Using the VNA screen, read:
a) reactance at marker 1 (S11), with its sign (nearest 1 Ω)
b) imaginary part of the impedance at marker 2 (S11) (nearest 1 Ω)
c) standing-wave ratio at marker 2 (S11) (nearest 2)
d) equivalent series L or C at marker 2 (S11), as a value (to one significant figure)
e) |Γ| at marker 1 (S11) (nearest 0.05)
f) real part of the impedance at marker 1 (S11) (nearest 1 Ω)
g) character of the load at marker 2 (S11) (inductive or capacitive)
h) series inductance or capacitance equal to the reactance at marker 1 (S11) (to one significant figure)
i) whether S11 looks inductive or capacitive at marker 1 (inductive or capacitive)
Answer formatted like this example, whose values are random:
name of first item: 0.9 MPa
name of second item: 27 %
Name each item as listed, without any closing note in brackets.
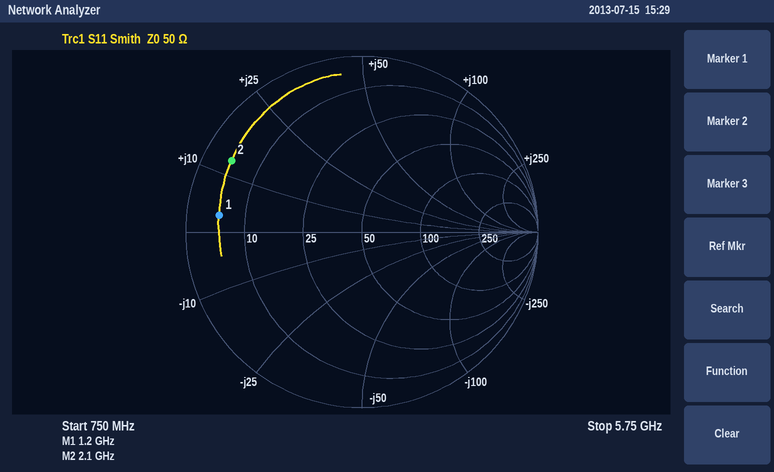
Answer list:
reactance at marker 1 (S11), with its sign: +3 Ω
imaginary part of the impedance at marker 2 (S11): +13 Ω
standing-wave ratio at marker 2 (S11): 12
equivalent series L or C at marker 2 (S11), as a value: 1.0 nH
|Γ| at marker 1 (S11): 0.80
real part of the impedance at marker 1 (S11): 5 Ω
character of the load at marker 2 (S11): inductive
series inductance or capacitance equal to the reactance at marker 1 (S11): 400 pH
whether S11 looks inductive or capacitive at marker 1: inductive
